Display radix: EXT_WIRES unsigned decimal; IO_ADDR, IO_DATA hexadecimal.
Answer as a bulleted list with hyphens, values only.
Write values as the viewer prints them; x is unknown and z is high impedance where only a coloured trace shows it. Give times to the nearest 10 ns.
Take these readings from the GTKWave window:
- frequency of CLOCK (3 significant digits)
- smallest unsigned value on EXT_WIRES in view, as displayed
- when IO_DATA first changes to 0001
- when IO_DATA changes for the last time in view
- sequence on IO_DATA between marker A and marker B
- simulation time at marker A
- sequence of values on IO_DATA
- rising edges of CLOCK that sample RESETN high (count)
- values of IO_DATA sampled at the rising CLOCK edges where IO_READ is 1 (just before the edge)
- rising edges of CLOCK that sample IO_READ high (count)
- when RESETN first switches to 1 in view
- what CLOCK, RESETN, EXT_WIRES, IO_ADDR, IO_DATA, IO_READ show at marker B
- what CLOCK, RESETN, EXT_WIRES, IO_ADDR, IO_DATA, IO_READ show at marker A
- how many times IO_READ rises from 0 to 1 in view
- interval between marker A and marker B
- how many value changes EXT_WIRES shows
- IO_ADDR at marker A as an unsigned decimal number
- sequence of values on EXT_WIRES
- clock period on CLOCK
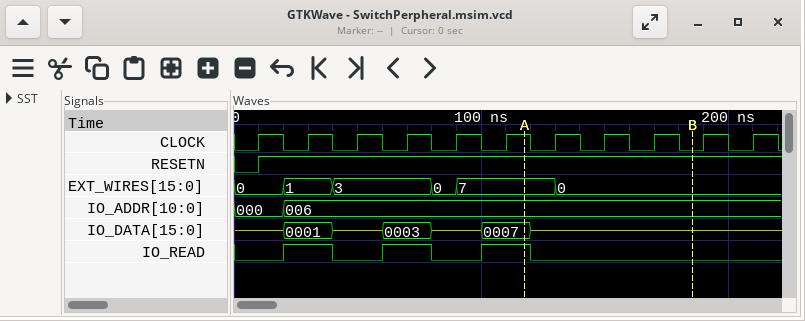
- 50.0 MHz
- 0
- 20 ns
- 120 ns
- 0007, z
- 120 ns
- z, 0001, z, 0003, z, 0007, z
- 10
- 0001, 0003, 0007
- 3
- 10 ns
- CLOCK=0, RESETN=1, EXT_WIRES=0, IO_ADDR=006, IO_DATA=z, IO_READ=0
- CLOCK=1, RESETN=1, EXT_WIRES=7, IO_ADDR=006, IO_DATA=0007, IO_READ=1
- 3
- 70 ns
- 5
- 6
- 0, 1, 3, 0, 7, 0
- 20 ns
